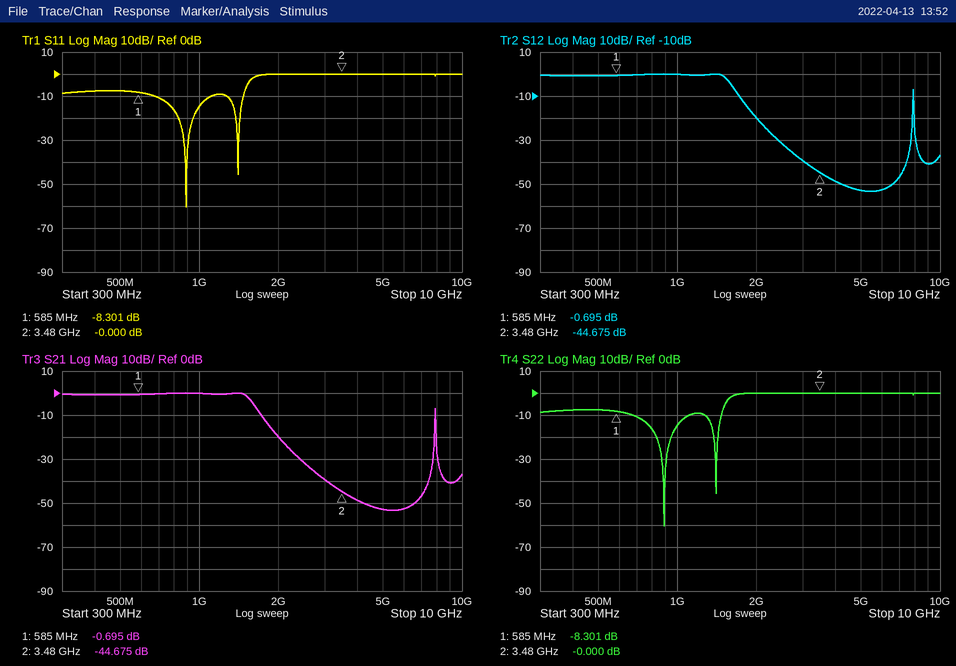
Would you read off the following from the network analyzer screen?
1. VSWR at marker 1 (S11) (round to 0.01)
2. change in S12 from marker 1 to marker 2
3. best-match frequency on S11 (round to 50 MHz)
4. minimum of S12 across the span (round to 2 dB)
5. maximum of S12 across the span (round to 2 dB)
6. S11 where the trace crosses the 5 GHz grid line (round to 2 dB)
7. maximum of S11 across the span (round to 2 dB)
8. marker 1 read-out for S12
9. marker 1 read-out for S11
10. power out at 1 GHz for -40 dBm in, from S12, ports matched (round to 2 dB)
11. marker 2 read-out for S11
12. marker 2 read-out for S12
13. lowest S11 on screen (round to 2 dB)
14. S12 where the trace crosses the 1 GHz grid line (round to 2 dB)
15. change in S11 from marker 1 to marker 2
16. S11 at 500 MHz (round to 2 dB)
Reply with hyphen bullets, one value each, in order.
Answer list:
- 2.25
- -43.980 dB
- 900 MHz
- -54 dB
- 0 dB
- 0 dB
- 0 dB
- -0.695 dB
- -8.301 dB
- -40 dBm
- -0.000 dB
- -44.675 dB
- -60 dB
- 0 dB
- 8.301 dB
- -8 dB
